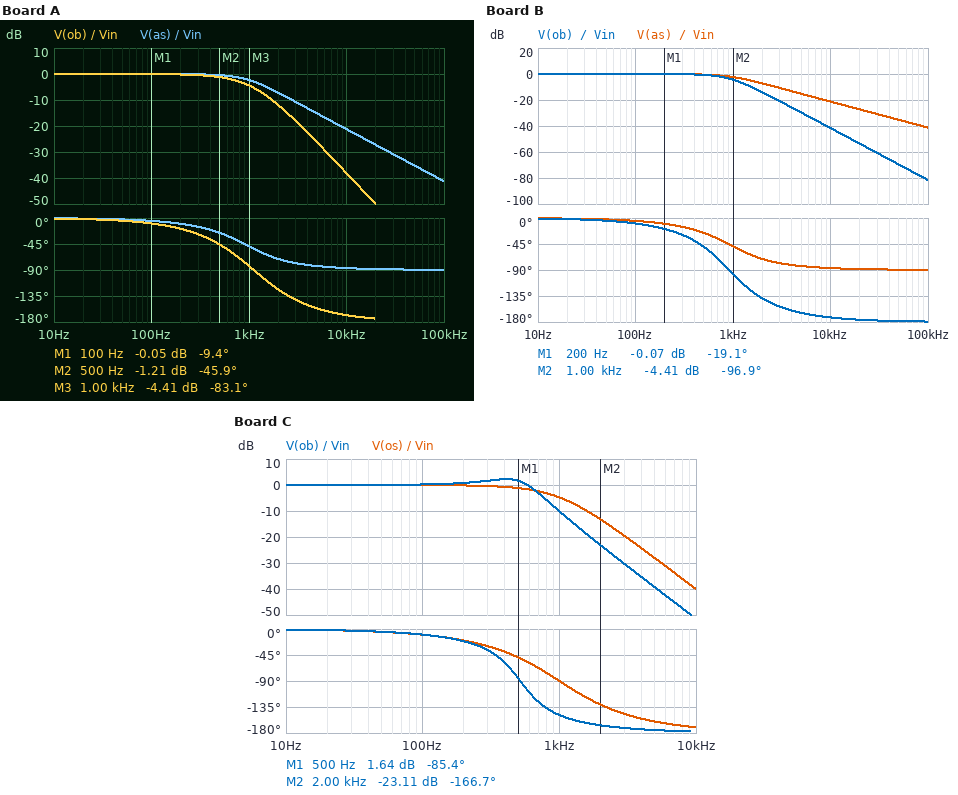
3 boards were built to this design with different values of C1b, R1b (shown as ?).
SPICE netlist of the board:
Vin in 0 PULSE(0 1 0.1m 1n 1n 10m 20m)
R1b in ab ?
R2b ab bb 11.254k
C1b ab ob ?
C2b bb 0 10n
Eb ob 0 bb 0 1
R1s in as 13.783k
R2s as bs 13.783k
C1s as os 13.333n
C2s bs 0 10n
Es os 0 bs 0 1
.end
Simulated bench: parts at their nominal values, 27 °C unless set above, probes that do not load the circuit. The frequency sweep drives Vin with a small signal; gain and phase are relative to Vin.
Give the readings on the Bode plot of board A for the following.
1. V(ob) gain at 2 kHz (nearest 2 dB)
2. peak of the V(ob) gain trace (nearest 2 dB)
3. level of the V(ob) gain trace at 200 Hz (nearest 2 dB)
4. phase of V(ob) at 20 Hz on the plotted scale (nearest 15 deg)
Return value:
-12 dB
0 dB
0 dB
0 deg
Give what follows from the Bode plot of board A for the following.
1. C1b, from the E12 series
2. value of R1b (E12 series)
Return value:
12 nF
15 kΩ
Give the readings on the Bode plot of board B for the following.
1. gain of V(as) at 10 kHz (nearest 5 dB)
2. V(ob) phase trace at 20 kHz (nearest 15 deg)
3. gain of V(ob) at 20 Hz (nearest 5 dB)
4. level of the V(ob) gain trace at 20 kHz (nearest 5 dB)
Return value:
-20 dB
-180 deg
0 dB
-55 dB
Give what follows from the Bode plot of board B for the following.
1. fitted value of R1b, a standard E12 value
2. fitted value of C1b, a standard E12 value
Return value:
15 kΩ
18 nF
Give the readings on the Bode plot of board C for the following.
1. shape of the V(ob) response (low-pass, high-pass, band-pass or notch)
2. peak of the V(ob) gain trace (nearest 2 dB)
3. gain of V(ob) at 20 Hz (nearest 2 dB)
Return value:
low-pass
2 dB
0 dB
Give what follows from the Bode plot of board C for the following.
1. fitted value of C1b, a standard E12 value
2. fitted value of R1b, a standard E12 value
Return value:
56 nF
15 kΩ
